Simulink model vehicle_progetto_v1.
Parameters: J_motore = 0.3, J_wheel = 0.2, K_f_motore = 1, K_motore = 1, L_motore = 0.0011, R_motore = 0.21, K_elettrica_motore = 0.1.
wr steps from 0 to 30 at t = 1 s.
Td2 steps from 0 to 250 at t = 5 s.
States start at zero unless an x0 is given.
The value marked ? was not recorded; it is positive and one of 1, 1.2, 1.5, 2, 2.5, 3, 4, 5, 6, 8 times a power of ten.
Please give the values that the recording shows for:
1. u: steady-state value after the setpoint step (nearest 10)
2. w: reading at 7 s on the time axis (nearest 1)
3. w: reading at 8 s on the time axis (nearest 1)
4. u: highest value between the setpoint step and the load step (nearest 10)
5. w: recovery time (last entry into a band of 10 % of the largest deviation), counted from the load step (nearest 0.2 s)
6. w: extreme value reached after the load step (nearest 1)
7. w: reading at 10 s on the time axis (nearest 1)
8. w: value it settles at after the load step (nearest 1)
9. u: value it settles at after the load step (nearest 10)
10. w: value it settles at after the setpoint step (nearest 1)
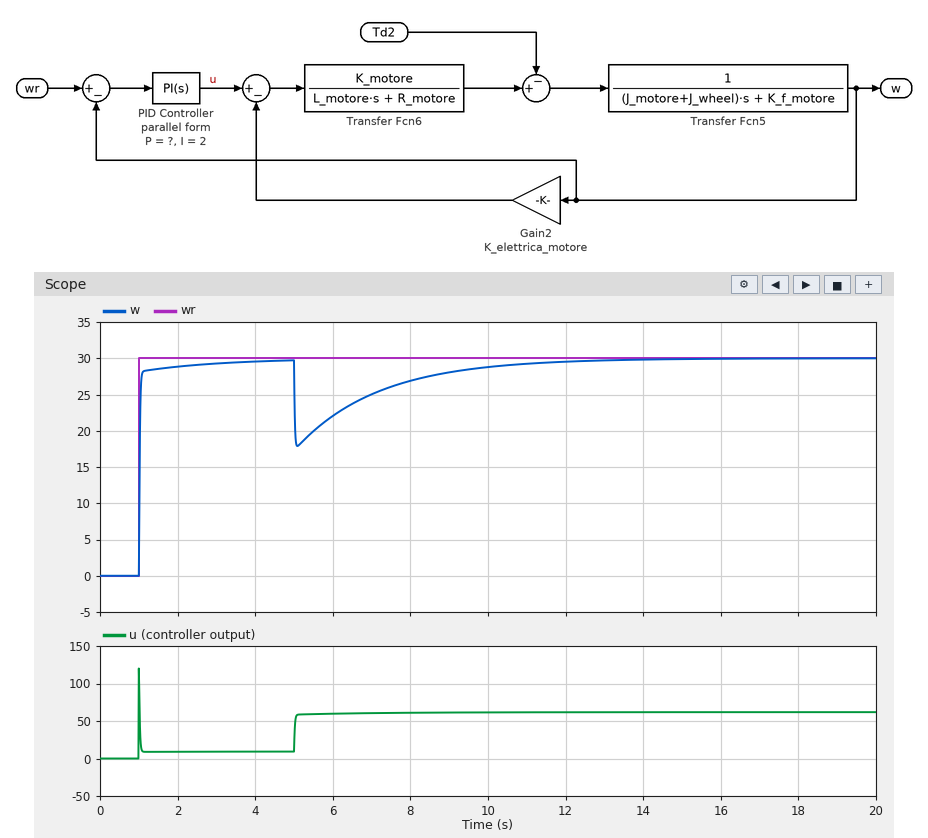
10
25
27
120
5.0 s
18
29
30
60
30
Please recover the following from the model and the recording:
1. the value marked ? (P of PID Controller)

4
